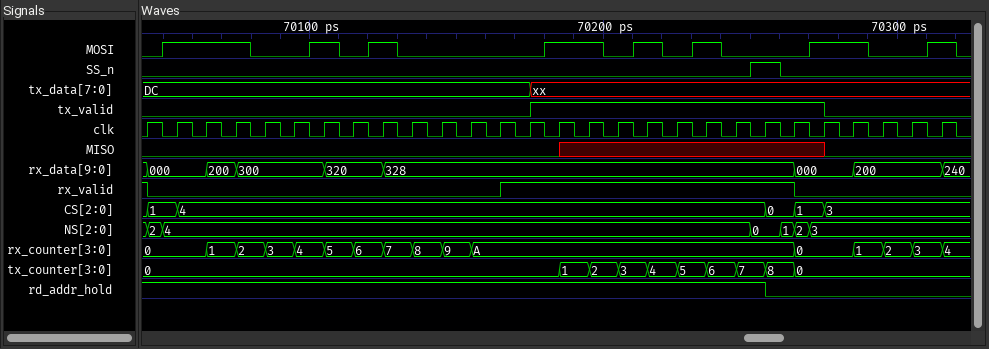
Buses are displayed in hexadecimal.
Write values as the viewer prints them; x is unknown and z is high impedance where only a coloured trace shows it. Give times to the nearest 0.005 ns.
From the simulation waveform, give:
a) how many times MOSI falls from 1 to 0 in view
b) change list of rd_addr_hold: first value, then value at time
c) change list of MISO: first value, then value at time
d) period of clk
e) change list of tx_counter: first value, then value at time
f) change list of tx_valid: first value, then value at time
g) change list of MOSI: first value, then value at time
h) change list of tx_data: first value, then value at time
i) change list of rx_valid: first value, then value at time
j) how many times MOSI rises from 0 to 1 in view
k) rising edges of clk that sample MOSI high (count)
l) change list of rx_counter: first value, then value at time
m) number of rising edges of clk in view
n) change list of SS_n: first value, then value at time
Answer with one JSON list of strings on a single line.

["8", "1, 0 at 70.255 ns", "0, x at 70.185 ns, 0 at 70.275 ns", "0.01 ns", "0, 1 at 70.185 ns, 2 at 70.195 ns, 3 at 70.205 ns, 4 at 70.215 ns, 5 at 70.225 ns, 6 at 70.235 ns, 7 at 70.245 ns, 8 at 70.255 ns, 0 at 70.265 ns", "0, 1 at 70.175 ns, 0 at 70.275 ns", "0, 1 at 70.05 ns, 0 at 70.08 ns, 1 at 70.1 ns, 0 at 70.11 ns, 1 at 70.12 ns, 0 at 70.13 ns, 1 at 70.18 ns, 0 at 70.2 ns, 1 at 70.21 ns, 0 at 70.22 ns, 1 at 70.23 ns, 0 at 70.24 ns, 1 at 70.27 ns, 0 at 70.29 ns, 1 at 70.31 ns, 0 at 70.32 ns", "DC, xx at 70.175 ns", "1, 0 at 70.045 ns, 1 at 70.165 ns, 0 at 70.265 ns", "8", "12", "0, 1 at 70.065 ns, 2 at 70.075 ns, 3 at 70.085 ns, 4 at 70.095 ns, 5 at 70.105 ns, 6 at 70.115 ns, 7 at 70.125 ns, 8 at 70.135 ns, 9 at 70.145 ns, A at 70.155 ns, 0 at 70.265 ns, 1 at 70.285 ns, 2 at 70.295 ns, 3 at 70.305 ns, 4 at 70.315 ns", "28", "0, 1 at 70.25 ns, 0 at 70.26 ns"]
